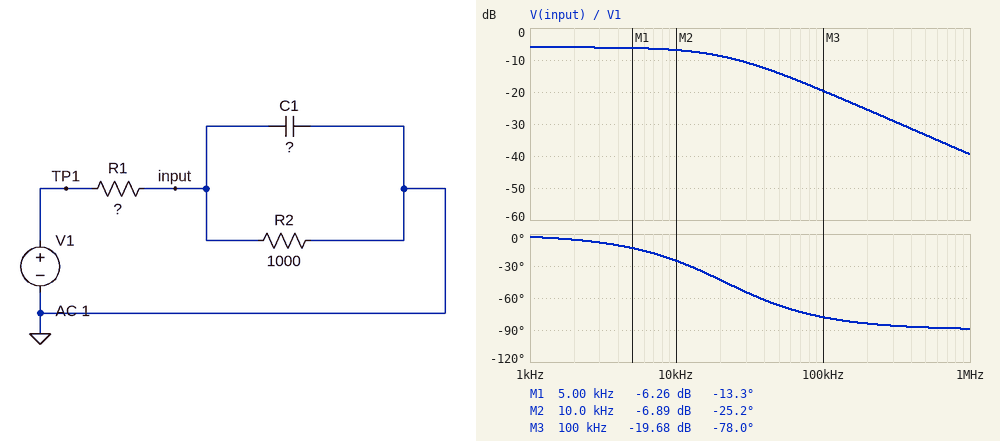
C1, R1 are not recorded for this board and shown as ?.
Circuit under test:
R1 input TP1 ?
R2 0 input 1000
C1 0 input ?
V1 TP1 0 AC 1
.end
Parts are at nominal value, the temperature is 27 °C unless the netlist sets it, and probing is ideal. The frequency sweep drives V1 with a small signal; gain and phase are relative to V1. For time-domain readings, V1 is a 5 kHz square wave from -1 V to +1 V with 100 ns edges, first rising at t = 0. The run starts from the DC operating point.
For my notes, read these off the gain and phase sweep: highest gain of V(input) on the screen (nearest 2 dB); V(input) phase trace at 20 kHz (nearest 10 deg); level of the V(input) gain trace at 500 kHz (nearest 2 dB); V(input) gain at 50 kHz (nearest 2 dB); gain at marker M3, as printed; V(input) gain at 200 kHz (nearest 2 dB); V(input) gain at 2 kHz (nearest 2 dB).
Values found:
-6 dB
-40 deg
-34 dB
-14 dB
-19.68 dB
-26 dB
-6 dB
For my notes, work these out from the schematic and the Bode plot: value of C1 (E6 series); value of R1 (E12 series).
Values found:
15 nF
1 kΩ
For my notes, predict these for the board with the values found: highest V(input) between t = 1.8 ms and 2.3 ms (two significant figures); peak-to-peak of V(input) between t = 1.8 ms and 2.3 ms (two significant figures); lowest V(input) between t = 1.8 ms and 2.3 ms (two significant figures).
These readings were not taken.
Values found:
500 mV
1.0 V
-500 mV
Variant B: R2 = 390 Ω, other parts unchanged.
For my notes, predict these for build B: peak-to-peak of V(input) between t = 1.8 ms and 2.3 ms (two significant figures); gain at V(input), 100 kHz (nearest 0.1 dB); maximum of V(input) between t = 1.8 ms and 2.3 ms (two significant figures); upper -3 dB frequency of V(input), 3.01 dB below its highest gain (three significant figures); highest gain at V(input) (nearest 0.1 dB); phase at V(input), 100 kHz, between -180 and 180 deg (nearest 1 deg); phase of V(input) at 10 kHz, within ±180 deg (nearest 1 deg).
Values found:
560 mV
-20.1 dB
280 mV
37.8 kHz
-11.0 dB
-69 deg
-15 deg
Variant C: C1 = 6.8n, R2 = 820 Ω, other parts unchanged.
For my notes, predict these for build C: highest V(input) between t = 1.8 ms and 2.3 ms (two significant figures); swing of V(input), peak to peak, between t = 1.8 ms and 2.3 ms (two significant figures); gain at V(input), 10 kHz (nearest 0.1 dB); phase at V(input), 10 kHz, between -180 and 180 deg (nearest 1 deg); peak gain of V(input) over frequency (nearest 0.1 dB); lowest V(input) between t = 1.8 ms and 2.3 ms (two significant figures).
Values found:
450 mV
900 mV
-7.1 dB
-11 deg
-6.9 dB
-450 mV
